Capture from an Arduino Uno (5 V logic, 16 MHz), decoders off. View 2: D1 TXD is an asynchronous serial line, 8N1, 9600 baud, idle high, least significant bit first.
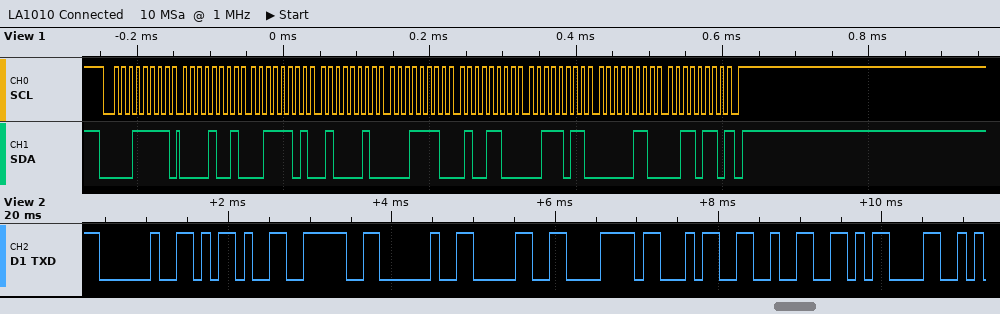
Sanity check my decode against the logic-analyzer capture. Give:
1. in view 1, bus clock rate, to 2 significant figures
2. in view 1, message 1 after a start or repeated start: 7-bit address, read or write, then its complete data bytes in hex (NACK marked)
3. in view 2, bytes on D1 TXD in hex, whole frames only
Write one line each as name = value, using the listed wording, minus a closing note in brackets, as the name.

in view 1, bus clock rate, to 2 significant figures = 100 kHz
in view 1, message 1 after a start or repeated start: 7-bit address, read or write, then its complete data bytes in hex = 0x0F read: 09 3D 42 1E 4C 3B 06 36 NACK
in view 2, bytes on D1 TXD in hex, whole frames only = 20 2D 3E 20 30 78 34 32 0D
